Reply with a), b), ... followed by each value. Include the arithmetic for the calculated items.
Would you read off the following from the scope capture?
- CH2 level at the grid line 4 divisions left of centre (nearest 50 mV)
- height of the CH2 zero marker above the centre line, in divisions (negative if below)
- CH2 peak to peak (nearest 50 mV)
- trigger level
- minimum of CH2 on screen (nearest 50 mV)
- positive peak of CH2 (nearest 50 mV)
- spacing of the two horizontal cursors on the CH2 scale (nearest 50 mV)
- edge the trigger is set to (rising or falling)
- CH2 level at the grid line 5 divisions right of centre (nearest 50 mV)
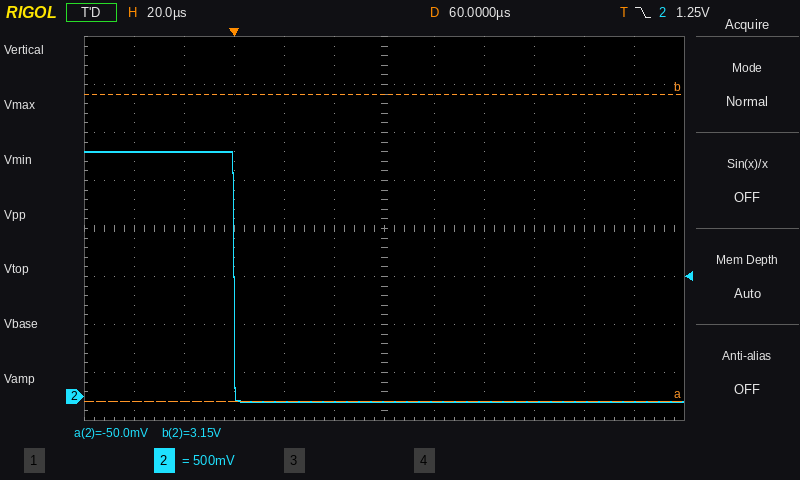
a) 2.55 V
b) -3.5 div
c) 2.55 V − (-50 mV) = 2.60 V
d) 1.25 V
e) -50 mV
f) 2.55 V
g) 3.20 V
h) falling
i) -50 mV
